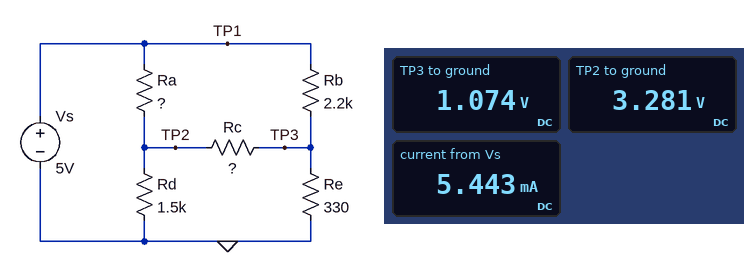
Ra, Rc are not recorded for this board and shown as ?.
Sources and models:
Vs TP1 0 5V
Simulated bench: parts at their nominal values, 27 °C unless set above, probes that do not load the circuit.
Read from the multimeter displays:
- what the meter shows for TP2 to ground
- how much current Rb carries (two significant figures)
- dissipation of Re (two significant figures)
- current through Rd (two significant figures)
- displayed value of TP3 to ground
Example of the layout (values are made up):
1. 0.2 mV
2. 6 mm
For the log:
1. 3.281 V
2. 1.8 mA
3. 3.5 mW
4. 2.2 mA
5. 1.074 V
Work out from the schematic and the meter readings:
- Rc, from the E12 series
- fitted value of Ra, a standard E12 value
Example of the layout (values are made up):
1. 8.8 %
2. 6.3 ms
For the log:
1. 1.5 kΩ
2. 470 Ω
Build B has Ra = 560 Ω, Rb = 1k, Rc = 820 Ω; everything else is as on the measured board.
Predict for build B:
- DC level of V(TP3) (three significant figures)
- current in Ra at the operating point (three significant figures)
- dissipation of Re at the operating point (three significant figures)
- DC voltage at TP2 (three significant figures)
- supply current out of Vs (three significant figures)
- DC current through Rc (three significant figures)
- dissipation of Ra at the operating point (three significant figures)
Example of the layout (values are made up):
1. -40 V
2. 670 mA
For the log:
1. 1.64 V
2. 3.61 mA
3. 8.19 mW
4. 2.98 V
5. 6.97 mA
6. 1.63 mA
7. 7.30 mW
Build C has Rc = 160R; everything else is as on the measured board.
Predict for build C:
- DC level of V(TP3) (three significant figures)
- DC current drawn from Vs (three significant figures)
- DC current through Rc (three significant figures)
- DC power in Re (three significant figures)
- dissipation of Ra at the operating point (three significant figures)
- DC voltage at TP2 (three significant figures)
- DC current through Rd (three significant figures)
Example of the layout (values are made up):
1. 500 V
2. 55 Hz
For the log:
1. 1.78 V
2. 6.99 mA
3. 3.92 mA
4. 9.57 mW
5. 14.3 mW
6. 2.40 V
7. 1.60 mA
